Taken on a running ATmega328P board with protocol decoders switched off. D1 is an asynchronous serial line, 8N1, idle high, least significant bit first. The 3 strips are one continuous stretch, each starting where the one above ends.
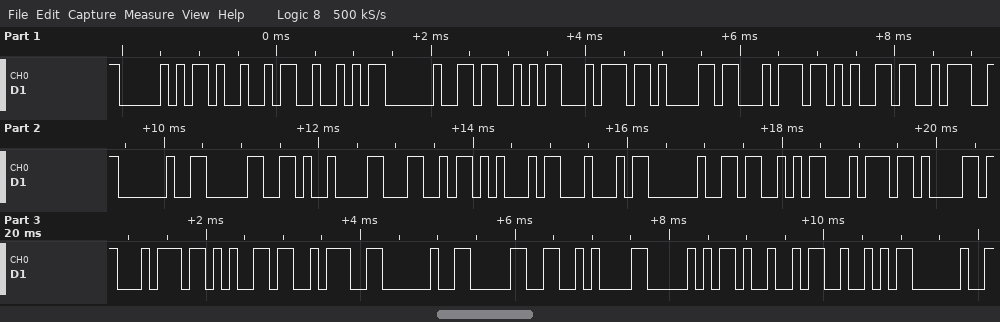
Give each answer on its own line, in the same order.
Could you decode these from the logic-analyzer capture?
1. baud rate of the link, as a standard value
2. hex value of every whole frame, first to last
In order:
9600 baud
50 49 52 20 53 74 61 74 65 3A 20 30 09 4C 45 44 20 53 74 61 74 65 3A 20 30 0A 50 49 52 20
